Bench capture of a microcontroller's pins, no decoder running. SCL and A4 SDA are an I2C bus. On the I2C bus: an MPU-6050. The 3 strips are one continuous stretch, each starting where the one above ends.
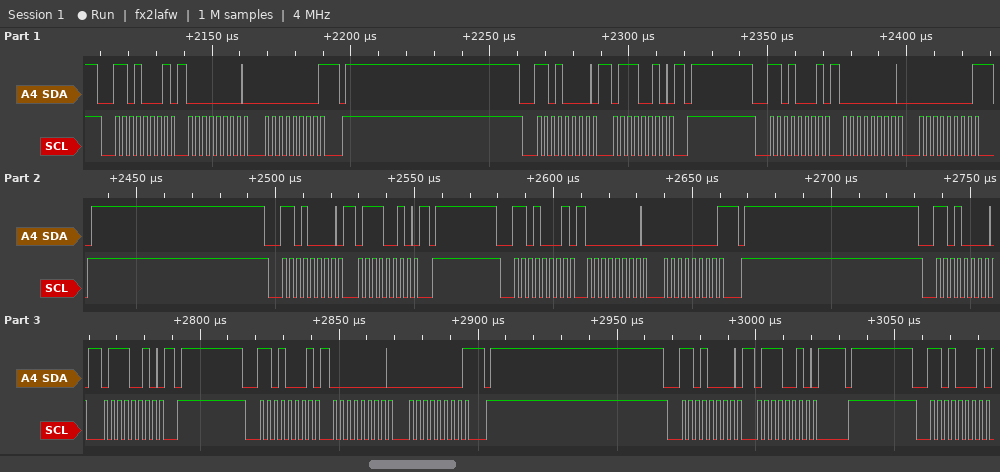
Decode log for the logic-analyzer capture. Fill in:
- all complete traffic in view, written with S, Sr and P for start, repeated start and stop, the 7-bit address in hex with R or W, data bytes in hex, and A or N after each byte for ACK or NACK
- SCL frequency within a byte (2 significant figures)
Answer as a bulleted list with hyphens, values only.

- S 68R A 00 A 00 N P S 68W A 72 A P S 68R A 00 A 00 N P S 68W A 72 A P S 68R A 00 A 00 N P S 68W A 72 A P S 68R A 00 A 00 N P S 68W A 72 A P S 68R A
- 400 kHz
